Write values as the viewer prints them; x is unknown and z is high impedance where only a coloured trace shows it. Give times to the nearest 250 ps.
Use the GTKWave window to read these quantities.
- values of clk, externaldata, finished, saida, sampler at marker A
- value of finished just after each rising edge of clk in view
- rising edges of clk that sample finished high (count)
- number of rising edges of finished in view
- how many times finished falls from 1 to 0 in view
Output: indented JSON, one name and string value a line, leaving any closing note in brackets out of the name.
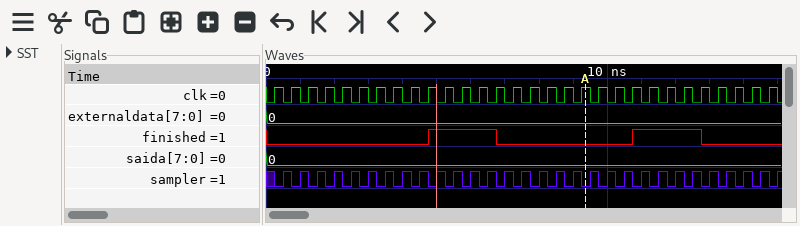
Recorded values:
{
  "values of clk, externaldata, finished, saida, sampler at marker A": "clk=1, externaldata=0, finished=0, saida=0, sampler=0",
  "value of finished just after each rising edge of clk in view": "0 0 0 0 0 0 0 0 0 1 1 1 1 0 0 0 0 0 0 0 0 1 1 1 1 0 0 0 0 0",
  "rising edges of clk that sample finished high": "8",
  "number of rising edges of finished in view": "2",
  "how many times finished falls from 1 to 0 in view": "2"
}
